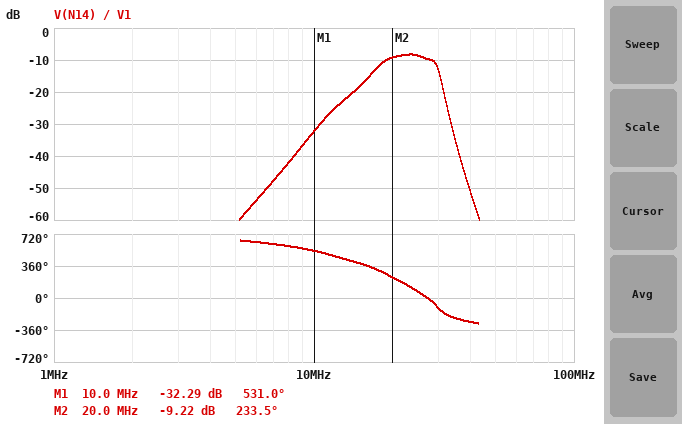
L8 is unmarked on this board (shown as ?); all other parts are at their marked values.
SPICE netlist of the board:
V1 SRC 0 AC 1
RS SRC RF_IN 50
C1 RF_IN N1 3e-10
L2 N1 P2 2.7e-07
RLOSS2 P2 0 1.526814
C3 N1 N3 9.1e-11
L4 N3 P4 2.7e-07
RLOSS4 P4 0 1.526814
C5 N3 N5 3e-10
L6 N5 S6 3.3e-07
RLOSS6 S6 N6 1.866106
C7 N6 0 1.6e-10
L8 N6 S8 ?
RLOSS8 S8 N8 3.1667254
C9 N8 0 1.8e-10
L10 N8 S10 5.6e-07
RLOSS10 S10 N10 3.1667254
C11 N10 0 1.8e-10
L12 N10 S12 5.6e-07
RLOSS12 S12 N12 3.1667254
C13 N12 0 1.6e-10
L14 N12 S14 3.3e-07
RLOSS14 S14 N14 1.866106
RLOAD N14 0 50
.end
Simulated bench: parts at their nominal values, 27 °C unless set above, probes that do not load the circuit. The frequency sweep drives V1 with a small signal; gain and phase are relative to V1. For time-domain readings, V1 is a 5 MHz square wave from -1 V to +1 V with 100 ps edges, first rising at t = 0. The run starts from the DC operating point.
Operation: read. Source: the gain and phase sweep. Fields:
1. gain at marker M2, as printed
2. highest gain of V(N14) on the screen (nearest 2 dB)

-9.22 dB
-8 dB
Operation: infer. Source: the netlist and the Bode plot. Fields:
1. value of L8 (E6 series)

680 nH
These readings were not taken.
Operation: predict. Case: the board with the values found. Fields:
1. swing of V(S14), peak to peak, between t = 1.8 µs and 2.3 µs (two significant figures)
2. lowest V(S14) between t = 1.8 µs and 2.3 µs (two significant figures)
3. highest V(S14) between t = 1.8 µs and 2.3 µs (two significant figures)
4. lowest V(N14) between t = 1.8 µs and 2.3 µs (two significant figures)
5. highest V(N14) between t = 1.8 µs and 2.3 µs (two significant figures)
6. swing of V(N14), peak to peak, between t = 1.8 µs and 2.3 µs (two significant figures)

310 mV
-150 mV
150 mV
-150 mV
150 mV
300 mV
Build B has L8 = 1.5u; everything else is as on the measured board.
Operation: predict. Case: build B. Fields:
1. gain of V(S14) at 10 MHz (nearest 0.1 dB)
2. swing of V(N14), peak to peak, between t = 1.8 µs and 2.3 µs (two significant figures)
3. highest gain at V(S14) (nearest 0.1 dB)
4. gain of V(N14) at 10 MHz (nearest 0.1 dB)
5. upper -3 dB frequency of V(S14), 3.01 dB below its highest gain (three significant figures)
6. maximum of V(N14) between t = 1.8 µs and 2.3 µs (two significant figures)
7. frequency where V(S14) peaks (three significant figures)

-34.9 dB
130 mV
-9.3 dB
-35.2 dB
22.0 MHz
64 mV
19.4 MHz
